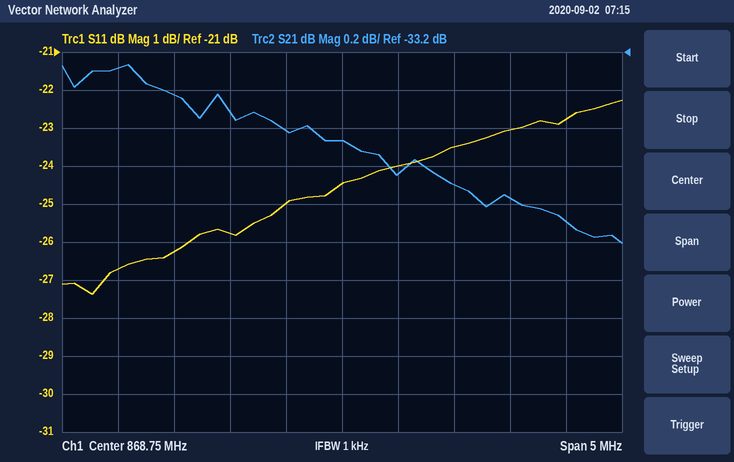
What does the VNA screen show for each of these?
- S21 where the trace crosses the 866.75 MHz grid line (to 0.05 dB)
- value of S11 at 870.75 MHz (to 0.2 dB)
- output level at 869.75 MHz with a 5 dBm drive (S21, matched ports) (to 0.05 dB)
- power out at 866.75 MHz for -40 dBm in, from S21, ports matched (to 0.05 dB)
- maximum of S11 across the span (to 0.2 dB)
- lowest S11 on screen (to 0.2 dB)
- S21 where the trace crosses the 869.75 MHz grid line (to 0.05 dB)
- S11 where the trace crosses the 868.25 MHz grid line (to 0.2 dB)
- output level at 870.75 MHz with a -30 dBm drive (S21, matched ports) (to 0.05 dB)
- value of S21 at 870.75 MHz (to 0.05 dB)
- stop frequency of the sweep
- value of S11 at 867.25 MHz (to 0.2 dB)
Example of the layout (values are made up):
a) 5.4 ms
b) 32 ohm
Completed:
a) -33.30 dB
b) -22.8 dB
c) -28.90 dBm
d) -73.30 dBm
e) -22.2 dB
f) -27.4 dB
g) -33.90 dB
h) -25.0 dB
i) -64.10 dBm
j) -34.10 dB
k) 871.25 MHz
l) -26.2 dB
